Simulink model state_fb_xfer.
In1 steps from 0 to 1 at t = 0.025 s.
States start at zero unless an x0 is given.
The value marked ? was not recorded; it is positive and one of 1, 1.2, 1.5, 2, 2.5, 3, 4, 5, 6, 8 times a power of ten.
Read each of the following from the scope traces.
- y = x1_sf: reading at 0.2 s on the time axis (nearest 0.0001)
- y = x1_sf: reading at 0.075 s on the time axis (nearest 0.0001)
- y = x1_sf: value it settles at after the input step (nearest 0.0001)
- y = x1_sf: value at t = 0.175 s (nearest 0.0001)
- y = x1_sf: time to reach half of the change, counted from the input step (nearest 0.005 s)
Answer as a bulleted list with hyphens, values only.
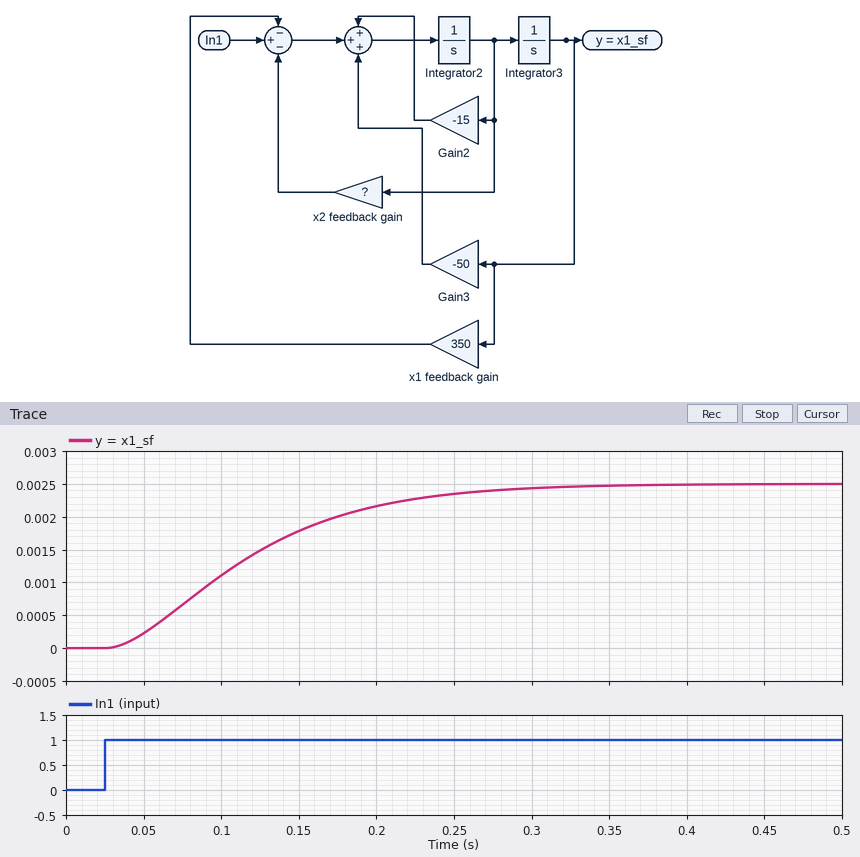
- 0.0022
- 0.0007
- 0.0025
- 0.0020
- 0.085 s
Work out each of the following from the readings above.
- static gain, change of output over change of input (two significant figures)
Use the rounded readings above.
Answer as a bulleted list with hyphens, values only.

- 0.0025
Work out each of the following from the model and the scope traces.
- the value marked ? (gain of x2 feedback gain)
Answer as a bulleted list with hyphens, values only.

- 25
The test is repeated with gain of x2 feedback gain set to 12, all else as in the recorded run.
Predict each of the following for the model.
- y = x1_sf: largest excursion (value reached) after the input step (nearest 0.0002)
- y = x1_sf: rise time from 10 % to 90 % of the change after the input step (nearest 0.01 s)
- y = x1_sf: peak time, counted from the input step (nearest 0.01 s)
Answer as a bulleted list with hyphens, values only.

- 0.0026
- 0.10 s
- 0.21 s
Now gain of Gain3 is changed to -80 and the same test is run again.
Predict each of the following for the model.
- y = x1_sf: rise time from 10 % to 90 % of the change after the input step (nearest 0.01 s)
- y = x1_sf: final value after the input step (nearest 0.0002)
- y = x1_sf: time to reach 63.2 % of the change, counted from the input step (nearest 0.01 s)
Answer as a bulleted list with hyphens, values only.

- 0.15 s
- 0.0024
- 0.10 s
